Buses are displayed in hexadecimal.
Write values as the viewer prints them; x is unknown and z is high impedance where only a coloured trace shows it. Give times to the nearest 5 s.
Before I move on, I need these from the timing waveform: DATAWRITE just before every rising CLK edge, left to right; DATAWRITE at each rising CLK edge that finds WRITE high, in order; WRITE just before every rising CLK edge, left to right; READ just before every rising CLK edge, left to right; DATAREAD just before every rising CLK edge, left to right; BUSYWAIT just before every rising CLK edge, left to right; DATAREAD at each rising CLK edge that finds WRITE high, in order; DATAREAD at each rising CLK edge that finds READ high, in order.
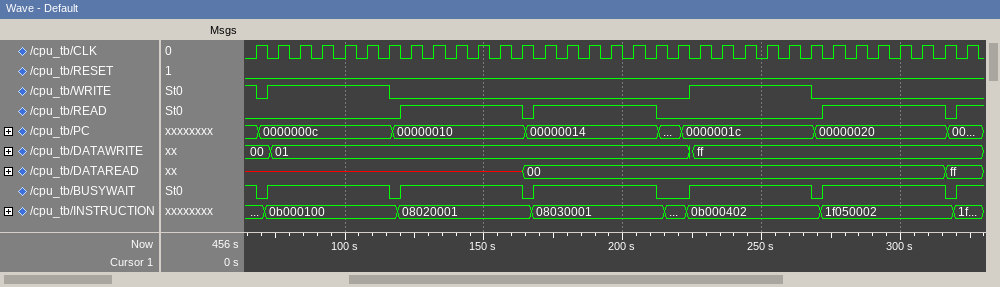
00, 01, 01, 01, 01, 01, 01, 01, 01, 01, 01, 01, 01, 01, 01, 01, 01, 01, 01, 01, ff, ff, ff, ff, ff, ff, ff, ff, ff, ff, ff, ff, ff
00, 01, 01, 01, 01, 01, 01, ff, ff, ff, ff, ff, ff
1 1 1 1 1 1 1 0 0 0 0 0 0 0 0 0 0 0 0 0 1 1 1 1 1 1 0 0 0 0 0 0 0
0 0 0 0 0 0 0 1 1 1 1 1 1 1 1 1 1 1 1 0 0 0 0 0 0 0 1 1 1 1 1 1 1
x, x, x, x, x, x, x, x, x, x, x, x, x, 00, 00, 00, 00, 00, 00, 00, 00, 00, 00, 00, 00, 00, 00, 00, 00, 00, 00, 00, ff
1 1 1 1 1 1 1 1 1 1 1 1 1 1 1 1 1 1 1 0 1 1 1 1 1 1 1 1 1 1 1 1 1
x, x, x, x, x, x, x, 00, 00, 00, 00, 00, 00
x, x, x, x, x, x, 00, 00, 00, 00, 00, 00, 00, 00, 00, 00, 00, 00, ff
